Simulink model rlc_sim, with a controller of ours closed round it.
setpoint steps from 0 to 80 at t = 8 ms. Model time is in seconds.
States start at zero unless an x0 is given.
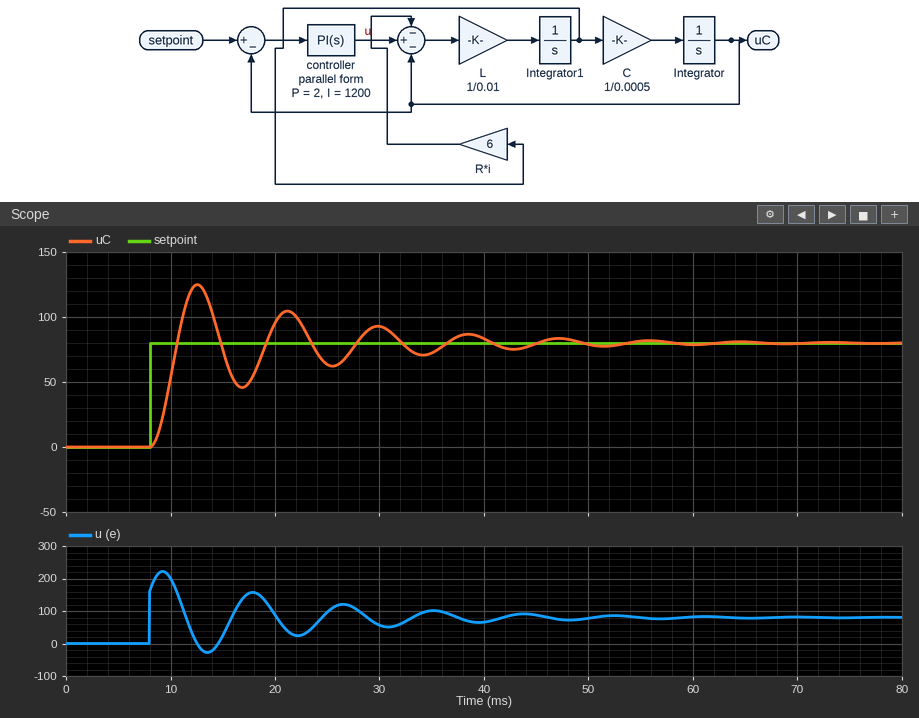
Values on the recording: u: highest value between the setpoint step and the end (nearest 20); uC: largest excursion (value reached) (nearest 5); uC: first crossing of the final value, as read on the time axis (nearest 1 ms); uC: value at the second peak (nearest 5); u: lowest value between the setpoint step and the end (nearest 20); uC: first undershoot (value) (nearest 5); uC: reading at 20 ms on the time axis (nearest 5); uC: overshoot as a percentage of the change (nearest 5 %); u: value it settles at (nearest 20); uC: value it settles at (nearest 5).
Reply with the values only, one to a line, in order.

220
125
11 ms
105
-20
45
95
55 %
80
80
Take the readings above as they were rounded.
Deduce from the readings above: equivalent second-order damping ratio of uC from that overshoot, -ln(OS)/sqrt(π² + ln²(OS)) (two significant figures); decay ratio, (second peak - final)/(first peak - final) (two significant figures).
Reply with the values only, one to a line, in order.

0.19
0.56
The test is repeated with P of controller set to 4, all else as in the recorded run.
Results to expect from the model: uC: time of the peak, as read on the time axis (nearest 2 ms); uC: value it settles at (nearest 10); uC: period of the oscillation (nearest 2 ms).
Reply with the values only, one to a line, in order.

12 ms
80
6 ms
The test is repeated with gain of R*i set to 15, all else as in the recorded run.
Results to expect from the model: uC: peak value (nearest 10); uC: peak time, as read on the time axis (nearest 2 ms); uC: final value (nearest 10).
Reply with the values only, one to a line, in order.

110
14 ms
80
